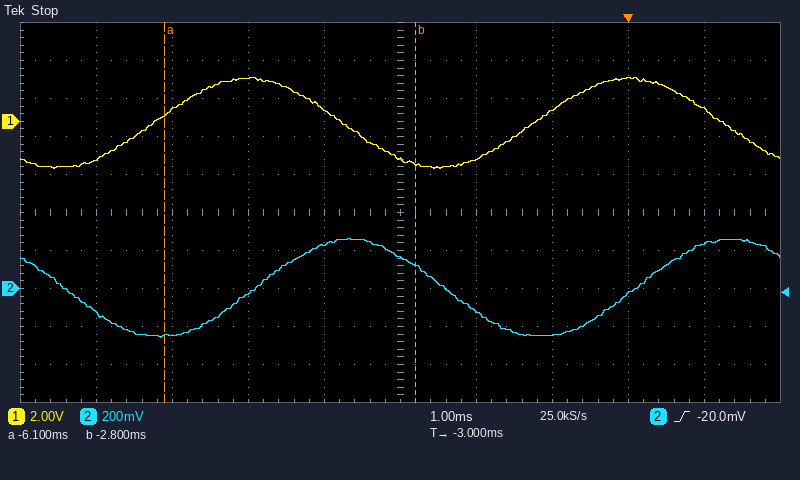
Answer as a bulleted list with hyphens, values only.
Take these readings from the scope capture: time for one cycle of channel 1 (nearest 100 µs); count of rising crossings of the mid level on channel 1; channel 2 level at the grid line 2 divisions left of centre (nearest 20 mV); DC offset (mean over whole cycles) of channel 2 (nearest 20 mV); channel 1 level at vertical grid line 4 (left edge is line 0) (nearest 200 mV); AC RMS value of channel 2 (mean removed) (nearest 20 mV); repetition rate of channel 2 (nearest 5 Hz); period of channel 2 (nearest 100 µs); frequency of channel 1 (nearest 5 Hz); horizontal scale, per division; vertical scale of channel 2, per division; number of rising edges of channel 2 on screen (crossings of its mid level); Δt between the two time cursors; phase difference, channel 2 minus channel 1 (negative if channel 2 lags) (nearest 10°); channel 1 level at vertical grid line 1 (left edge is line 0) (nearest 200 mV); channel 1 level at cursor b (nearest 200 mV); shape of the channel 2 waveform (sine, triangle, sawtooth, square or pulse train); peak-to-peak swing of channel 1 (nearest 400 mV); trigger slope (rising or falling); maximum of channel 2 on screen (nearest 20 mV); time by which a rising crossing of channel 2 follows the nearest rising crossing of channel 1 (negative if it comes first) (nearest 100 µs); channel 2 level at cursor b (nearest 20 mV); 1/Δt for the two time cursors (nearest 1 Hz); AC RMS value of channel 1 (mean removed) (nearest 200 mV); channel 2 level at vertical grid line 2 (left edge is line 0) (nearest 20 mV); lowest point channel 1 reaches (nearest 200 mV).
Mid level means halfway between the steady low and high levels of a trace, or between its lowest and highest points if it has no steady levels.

- 5.0 ms
- 2
- -20 mV
- 0 mV
- 600 mV
- 180 mV
- 200 Hz
- 5.0 ms
- 200 Hz
- 1 ms
- 200 mV
- 2
- 3.3 ms
- -100°
- -2.0 V
- -2.2 V
- sine
- 4.8 V
- rising
- 260 mV
- +1.4 ms
- 120 mV
- 303 Hz
- 1.6 V
- -240 mV
- -2.4 V
